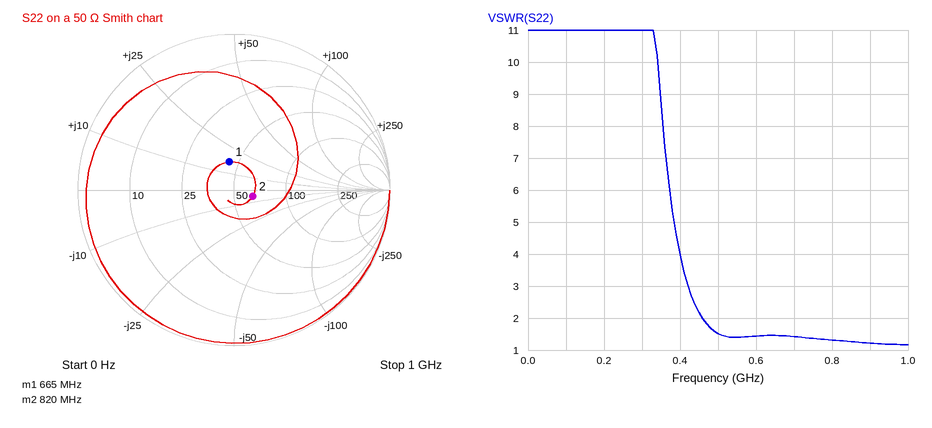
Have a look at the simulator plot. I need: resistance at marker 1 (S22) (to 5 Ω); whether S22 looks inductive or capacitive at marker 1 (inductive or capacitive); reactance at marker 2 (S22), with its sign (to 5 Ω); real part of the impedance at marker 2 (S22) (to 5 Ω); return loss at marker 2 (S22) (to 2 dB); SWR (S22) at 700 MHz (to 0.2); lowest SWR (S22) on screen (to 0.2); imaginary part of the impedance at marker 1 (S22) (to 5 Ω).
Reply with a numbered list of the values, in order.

1. 45 Ω
2. inductive
3. -5 Ω
4. 65 Ω
5. 18 dB
6. 1.4
7. 1.2
8. +15 Ω
